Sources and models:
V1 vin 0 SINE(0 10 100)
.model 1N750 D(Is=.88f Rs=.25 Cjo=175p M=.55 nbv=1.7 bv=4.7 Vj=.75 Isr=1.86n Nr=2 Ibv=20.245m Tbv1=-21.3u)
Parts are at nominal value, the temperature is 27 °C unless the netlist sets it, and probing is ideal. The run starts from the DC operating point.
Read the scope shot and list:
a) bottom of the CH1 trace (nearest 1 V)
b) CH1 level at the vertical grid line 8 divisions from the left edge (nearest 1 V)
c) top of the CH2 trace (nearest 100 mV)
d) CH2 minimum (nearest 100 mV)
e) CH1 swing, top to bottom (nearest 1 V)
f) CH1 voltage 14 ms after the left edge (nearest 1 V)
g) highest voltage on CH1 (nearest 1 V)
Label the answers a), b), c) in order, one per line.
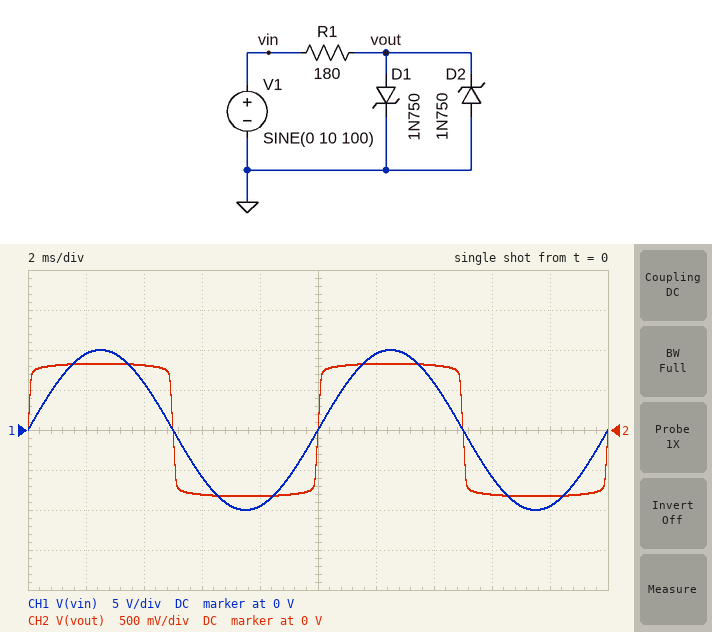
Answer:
a) -10 V
b) -6 V
c) 800 mV
d) -800 mV
e) 20 V
f) 6 V
g) 10 V
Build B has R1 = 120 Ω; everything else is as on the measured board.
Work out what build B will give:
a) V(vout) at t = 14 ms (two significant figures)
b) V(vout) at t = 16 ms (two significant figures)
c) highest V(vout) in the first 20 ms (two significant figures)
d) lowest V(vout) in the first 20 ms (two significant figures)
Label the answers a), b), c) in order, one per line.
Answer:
a) 820 mV
b) -820 mV
c) 850 mV
d) -850 mV
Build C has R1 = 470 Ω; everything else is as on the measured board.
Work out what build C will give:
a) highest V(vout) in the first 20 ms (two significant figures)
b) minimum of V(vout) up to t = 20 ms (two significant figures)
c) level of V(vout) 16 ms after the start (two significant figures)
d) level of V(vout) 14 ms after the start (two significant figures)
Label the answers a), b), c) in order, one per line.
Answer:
a) 800 mV
b) -800 mV
c) -780 mV
d) 780 mV
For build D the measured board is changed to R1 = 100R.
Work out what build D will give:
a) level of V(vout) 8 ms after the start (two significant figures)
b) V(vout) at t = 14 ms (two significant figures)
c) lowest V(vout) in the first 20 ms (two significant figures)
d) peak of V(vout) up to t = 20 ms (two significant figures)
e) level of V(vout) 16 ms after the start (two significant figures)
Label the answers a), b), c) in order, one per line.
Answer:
a) -850 mV
b) 830 mV
c) -860 mV
d) 860 mV
e) -830 mV
